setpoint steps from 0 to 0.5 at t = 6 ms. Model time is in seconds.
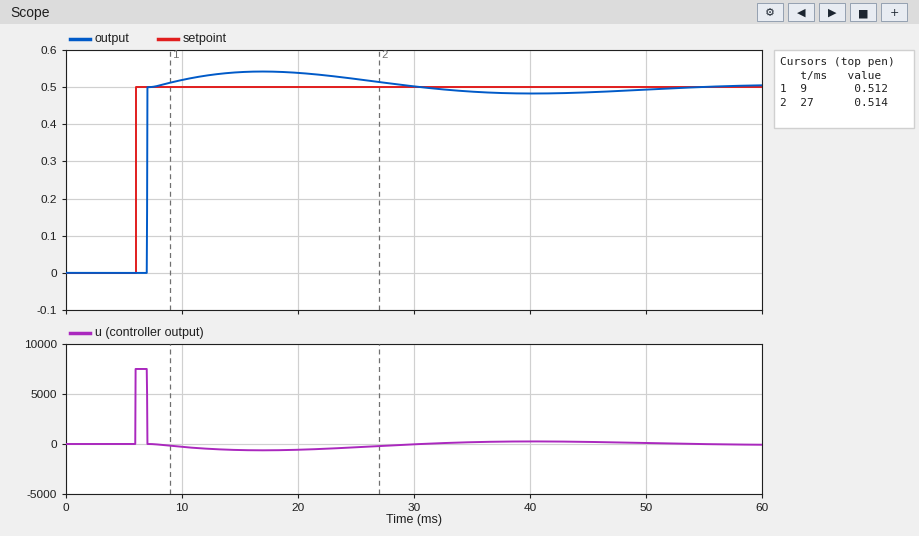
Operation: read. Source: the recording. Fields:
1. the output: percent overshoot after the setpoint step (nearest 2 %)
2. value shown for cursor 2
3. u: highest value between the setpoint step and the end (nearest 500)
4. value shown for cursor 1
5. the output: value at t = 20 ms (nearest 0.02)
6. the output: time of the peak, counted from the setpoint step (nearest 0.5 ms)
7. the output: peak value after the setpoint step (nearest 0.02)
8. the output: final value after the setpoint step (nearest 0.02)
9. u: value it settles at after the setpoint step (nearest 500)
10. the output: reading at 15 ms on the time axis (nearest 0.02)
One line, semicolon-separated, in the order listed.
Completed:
8 %; 0.514; 7500; 0.512; 0.54; 11.0 ms; 0.54; 0.50; 0; 0.54
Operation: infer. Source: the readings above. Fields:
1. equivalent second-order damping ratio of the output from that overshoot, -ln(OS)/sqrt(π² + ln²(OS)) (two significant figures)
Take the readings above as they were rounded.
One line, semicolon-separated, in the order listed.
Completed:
0.63
